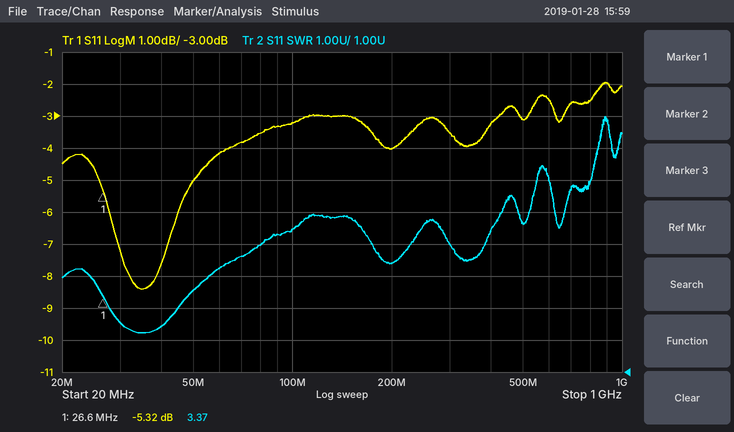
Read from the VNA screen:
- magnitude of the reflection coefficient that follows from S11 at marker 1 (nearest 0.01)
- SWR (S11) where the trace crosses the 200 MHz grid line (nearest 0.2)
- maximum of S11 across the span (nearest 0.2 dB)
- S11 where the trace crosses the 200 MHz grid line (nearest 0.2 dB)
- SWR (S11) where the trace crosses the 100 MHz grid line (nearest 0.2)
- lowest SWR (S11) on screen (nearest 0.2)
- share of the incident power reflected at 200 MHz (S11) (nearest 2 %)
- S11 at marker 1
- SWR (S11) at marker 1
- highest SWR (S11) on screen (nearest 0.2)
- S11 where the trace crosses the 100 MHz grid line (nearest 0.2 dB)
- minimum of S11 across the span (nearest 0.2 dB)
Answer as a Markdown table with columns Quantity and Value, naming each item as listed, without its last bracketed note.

| Quantity | Value |
|---|---|
| magnitude of the reflection coefficient that follows from S11 at marker 1 | 0.54 |
| SWR (S11) where the trace crosses the 200 MHz grid line | 4.4 |
| maximum of S11 across the span | -2.0 dB |
| S11 where the trace crosses the 200 MHz grid line | -4.0 dB |
| SWR (S11) where the trace crosses the 100 MHz grid line | 5.4 |
| lowest SWR (S11) on screen | 2.2 |
| share of the incident power reflected at 200 MHz (S11) | 40 % |
| S11 at marker 1 | -5.32 dB |
| SWR (S11) at marker 1 | 3.37 |
| highest SWR (S11) on screen | 9.0 |
| S11 where the trace crosses the 100 MHz grid line | -3.2 dB |
| minimum of S11 across the span | -8.4 dB |
